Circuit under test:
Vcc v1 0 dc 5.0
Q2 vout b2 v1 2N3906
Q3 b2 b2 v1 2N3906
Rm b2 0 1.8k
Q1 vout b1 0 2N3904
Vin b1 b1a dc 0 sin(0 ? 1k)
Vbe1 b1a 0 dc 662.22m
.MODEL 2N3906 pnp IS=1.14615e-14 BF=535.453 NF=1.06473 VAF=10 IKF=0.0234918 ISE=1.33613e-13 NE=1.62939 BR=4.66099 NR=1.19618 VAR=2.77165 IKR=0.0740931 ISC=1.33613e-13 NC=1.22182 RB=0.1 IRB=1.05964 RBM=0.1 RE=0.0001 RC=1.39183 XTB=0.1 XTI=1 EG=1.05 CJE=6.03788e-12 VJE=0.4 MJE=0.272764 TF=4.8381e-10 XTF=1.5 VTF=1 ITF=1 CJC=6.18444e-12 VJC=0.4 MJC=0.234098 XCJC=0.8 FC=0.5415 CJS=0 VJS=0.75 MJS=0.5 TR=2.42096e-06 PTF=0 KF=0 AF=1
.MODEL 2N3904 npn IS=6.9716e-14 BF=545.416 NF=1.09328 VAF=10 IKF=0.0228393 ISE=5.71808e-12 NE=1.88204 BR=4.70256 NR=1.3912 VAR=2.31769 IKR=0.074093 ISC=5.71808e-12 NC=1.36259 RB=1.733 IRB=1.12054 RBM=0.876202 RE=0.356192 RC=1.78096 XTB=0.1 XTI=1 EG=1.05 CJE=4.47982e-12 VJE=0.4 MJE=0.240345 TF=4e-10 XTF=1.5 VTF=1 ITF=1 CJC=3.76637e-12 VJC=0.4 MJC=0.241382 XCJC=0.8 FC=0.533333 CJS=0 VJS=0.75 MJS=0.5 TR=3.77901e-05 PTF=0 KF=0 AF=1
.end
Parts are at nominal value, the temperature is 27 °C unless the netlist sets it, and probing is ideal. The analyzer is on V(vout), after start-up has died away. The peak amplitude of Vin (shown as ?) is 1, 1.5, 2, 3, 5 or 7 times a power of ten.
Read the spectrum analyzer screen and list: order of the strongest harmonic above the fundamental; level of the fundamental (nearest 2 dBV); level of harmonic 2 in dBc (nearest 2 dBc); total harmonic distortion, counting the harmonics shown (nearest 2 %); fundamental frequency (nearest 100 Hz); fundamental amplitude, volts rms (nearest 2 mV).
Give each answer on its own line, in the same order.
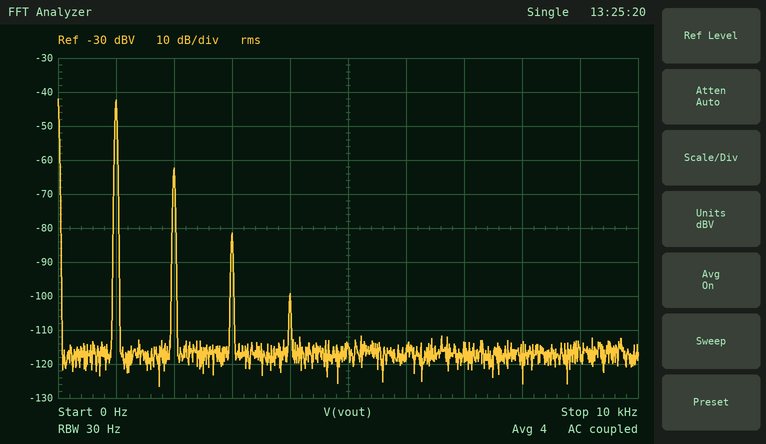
2
-42 dBV
-20 dBc
10 %
1.0 kHz
8 mV
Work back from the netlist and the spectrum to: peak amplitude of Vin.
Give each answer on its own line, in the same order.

7 mV
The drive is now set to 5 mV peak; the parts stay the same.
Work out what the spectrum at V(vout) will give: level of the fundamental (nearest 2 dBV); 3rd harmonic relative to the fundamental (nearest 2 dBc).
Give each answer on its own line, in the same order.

-46 dBV
-46 dBc
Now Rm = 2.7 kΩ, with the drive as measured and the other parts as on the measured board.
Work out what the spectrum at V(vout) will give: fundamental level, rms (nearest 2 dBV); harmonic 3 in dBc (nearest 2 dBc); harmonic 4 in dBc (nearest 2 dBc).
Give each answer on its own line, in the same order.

-32 dBV
-20 dBc
-28 dBc
